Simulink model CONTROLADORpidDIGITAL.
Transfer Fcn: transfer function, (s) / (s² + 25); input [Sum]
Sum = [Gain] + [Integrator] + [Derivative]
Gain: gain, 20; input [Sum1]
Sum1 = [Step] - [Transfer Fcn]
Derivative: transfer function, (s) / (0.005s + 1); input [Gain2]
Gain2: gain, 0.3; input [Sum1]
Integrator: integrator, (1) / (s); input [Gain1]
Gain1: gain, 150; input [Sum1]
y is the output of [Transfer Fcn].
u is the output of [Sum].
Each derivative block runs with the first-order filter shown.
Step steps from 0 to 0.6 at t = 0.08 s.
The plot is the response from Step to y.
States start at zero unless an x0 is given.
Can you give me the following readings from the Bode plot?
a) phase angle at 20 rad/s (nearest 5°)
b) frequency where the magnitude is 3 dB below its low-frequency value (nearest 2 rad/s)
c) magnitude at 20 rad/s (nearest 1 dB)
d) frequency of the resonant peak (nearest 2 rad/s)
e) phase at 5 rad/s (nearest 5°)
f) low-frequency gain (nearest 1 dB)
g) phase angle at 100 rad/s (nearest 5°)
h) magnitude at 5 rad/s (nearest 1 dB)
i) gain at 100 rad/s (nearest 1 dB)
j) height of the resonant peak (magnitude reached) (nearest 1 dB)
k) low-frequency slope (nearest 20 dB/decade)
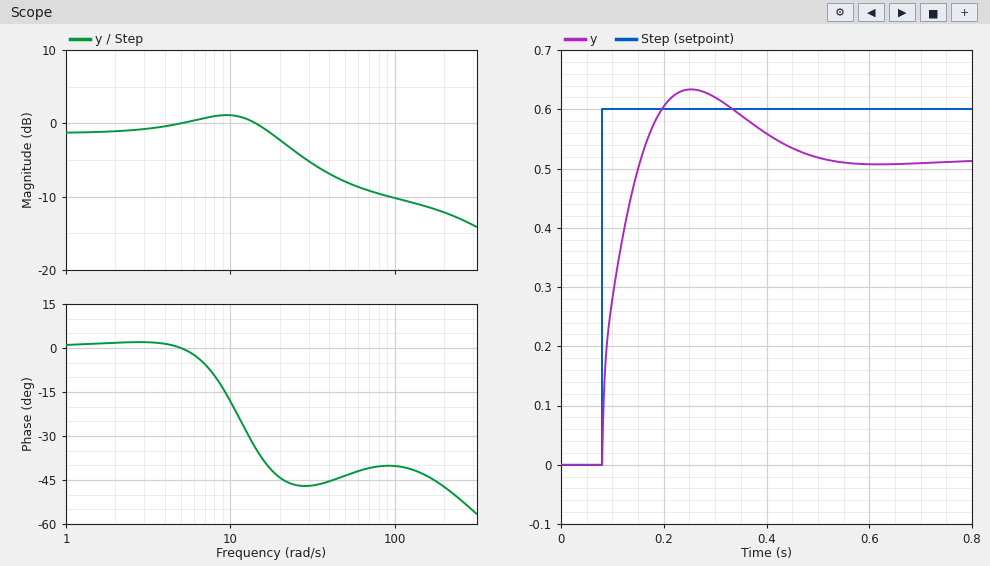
-45°
26 rad/s
-2 dB
10 rad/s
0°
-1 dB
-40°
0 dB
-10 dB
1 dB
0 dB/decade
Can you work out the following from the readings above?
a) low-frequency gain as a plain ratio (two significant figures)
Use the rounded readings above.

0.89
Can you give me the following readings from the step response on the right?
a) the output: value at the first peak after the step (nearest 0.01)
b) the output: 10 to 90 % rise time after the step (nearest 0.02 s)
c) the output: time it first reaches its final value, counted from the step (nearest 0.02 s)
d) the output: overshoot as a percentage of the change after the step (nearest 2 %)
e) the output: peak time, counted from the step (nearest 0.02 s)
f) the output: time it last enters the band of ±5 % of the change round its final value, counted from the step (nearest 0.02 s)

0.63
0.06 s
0.08 s
24 %
0.18 s
0.36 s
